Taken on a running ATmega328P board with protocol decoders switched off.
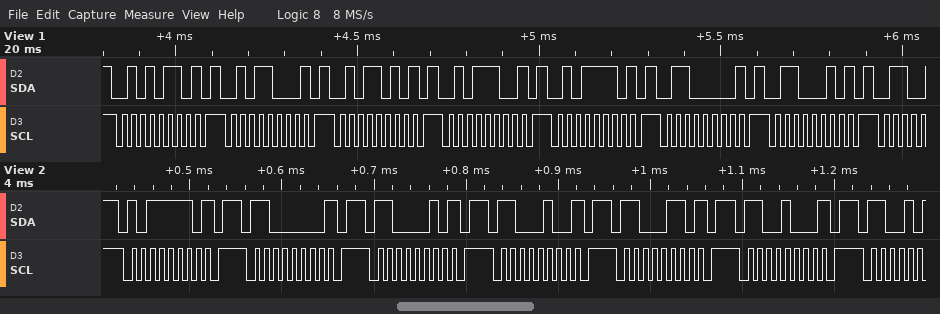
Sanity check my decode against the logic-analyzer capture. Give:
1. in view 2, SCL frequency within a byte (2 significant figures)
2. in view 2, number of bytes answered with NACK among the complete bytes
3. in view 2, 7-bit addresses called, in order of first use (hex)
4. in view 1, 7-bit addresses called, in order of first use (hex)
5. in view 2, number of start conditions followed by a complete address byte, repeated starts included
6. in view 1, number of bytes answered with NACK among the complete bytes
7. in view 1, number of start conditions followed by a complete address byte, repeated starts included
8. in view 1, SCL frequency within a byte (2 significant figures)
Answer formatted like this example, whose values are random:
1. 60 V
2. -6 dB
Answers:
1. 100 kHz
2. 6
3. 0x5F 0x60 0x61 0x62 0x63 0x64
4. 0x2B 0x2C 0x2D 0x2E 0x2F 0x30 0x31
5. 6
6. 7
7. 7
8. 40 kHz
